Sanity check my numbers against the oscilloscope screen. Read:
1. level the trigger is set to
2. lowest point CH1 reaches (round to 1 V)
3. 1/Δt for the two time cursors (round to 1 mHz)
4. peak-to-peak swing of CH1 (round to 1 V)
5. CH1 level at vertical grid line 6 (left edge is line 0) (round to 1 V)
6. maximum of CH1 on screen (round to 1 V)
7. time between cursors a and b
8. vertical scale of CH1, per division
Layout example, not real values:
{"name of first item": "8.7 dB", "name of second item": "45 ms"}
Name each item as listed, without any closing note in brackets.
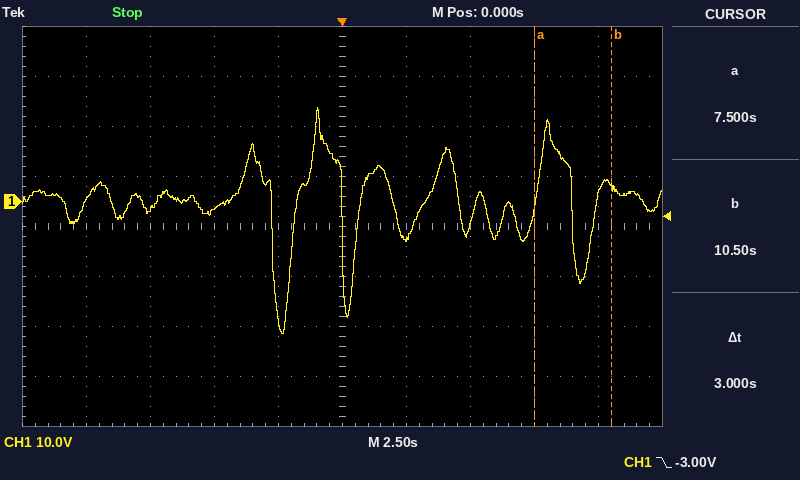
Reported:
{"level the trigger is set to": "-3.00 V", "lowest point CH1 reaches": "-26 V", "1/Δt for the two time cursors": "333 mHz", "peak-to-peak swing of CH1": "45 V", "CH1 level at vertical grid line 6 (left edge is line 0)": "-7 V", "maximum of CH1 on screen": "19 V", "time between cursors a and b": "3 s", "vertical scale of CH1, per division": "10 V"}
